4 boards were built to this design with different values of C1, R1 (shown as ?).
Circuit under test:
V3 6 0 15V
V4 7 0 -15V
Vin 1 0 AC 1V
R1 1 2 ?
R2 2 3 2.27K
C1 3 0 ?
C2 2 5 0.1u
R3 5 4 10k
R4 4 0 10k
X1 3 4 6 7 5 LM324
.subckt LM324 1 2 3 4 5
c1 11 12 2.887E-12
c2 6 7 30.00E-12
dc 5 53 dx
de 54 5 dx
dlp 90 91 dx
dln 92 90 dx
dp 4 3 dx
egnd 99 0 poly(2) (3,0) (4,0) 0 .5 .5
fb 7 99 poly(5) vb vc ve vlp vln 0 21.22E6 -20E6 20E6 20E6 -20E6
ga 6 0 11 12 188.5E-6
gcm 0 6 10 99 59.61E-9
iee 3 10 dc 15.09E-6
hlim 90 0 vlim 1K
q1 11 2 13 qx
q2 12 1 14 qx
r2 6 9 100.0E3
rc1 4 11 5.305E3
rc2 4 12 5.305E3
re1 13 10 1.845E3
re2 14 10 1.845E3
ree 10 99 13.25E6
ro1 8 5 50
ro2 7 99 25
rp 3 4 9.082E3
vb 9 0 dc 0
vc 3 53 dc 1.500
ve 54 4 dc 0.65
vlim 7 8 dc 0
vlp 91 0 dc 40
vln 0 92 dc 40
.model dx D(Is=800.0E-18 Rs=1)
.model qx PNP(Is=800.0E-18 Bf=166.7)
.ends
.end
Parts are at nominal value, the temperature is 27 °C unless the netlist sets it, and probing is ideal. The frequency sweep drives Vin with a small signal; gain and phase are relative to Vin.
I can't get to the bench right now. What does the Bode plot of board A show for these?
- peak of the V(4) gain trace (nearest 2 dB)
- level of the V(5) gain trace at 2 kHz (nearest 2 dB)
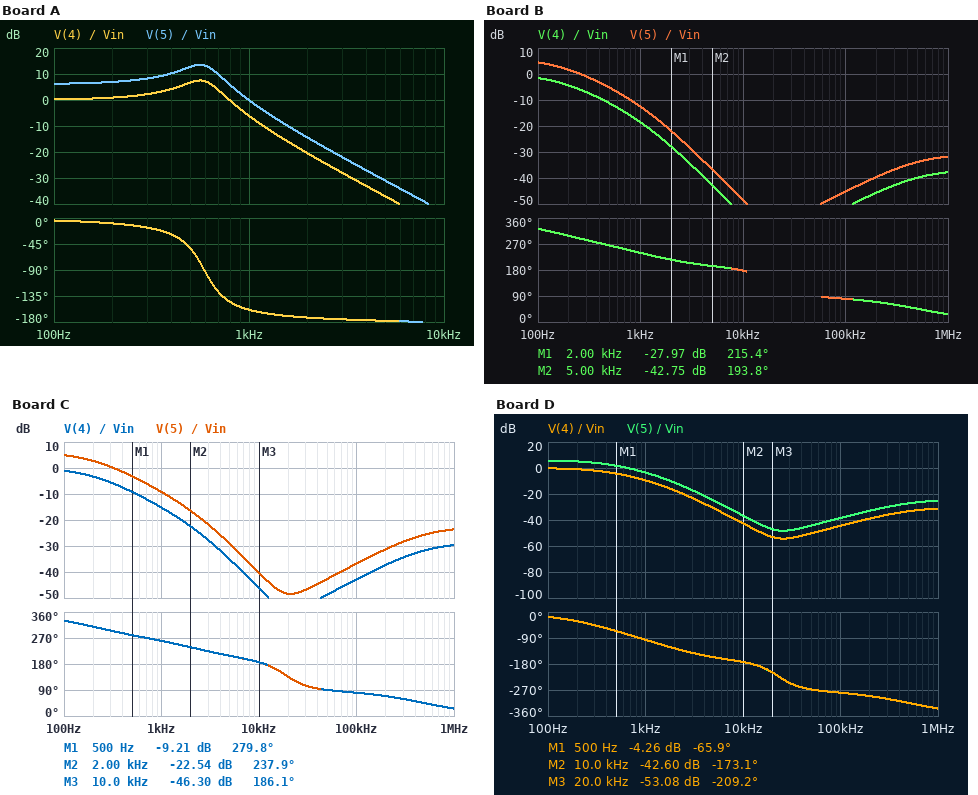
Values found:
8 dB
-14 dB
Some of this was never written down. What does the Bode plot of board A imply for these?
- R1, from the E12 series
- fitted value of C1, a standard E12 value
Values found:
3.9 kΩ
82 nF
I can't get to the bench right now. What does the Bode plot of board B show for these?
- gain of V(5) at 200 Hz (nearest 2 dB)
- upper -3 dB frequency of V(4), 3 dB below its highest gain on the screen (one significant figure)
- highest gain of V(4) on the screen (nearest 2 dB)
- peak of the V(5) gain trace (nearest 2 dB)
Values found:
2 dB
200 Hz
-2 dB
4 dB
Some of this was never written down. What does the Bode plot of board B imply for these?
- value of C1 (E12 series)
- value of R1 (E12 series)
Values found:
330 nF
1.8 kΩ
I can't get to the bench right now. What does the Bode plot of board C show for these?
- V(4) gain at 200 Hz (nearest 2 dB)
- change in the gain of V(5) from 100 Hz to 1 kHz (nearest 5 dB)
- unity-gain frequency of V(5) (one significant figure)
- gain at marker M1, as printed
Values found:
-4 dB
-15 dB
300 Hz
-9.21 dB
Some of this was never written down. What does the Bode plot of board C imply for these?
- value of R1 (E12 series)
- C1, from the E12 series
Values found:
680 Ω
330 nF
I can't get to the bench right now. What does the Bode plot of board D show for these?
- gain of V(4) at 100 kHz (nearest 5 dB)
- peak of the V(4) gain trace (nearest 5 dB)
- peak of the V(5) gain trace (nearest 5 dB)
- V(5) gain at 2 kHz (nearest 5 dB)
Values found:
-45 dB
0 dB
5 dB
-10 dB
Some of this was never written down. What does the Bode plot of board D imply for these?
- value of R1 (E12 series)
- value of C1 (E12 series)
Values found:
820 Ω
180 nF
